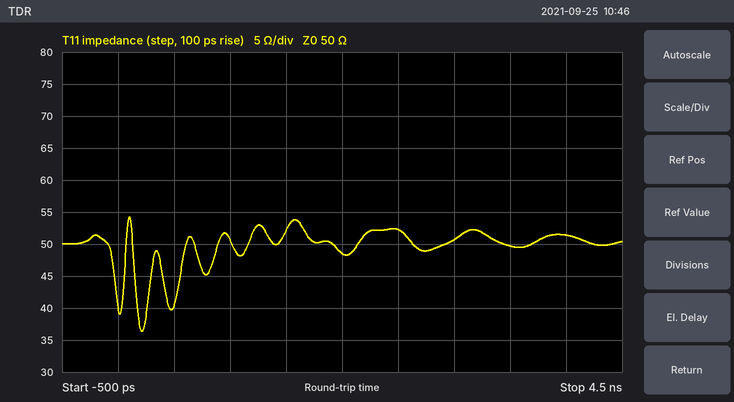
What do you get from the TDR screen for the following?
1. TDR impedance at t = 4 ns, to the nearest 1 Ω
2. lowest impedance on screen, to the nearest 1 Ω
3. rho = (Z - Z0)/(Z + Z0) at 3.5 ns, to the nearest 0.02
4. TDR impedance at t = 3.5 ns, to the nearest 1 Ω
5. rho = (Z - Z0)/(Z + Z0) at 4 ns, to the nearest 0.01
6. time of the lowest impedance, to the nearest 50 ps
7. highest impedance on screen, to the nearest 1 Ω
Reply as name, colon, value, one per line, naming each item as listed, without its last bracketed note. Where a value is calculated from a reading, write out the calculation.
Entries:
TDR impedance at t = 4 ns, to the nearest 1 Ω: 51 Ω
lowest impedance on screen, to the nearest 1 Ω: 36 Ω
rho = (Z - Z0)/(Z + Z0) at 3.5 ns, to the nearest 0.02: (50 − 50)/(50 + 50) ≈ 0.00
TDR impedance at t = 3.5 ns, to the nearest 1 Ω: 50 Ω
rho = (Z - Z0)/(Z + Z0) at 4 ns, to the nearest 0.01: (51 − 50)/(51 + 50) ≈ +0.01
time of the lowest impedance, to the nearest 50 ps: 200 ps
highest impedance on screen, to the nearest 1 Ω: 54 Ω
